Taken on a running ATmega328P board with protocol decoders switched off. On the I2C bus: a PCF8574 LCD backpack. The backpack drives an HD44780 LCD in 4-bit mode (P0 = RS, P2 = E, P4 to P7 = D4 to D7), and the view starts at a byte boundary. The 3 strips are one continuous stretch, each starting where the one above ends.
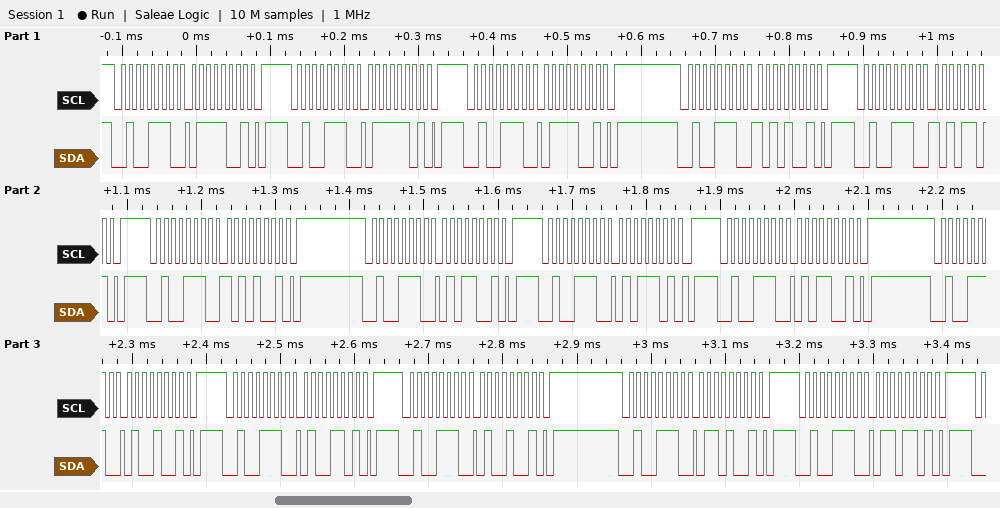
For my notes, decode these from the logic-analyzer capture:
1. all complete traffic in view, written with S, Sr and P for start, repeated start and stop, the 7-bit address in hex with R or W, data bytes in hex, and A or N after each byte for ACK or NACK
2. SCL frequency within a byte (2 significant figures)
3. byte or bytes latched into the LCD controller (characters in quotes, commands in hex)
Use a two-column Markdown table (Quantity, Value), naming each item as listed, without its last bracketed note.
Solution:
| Quantity | Value |
|---|---|
| all complete traffic in view, written with S, Sr and P for start, repeated start and stop, the 7-bit address in hex with R or W, data bytes in hex, and A or N after each byte for ACK or NACK | S 27W A 79 A P S 27W A 7D A P S 27W A 79 A P S 27W A A9 A P S 27W A AD A P S 27W A A9 A P S 27W A 59 A P S 27W A 5D A P S 27W A 59 A P S 27W A 49 A P S 27W A 4D A P S 27W A 49 A P S 27W A 69 A P S 27W A 6D A P |
| SCL frequency within a byte | 100 kHz |
| byte or bytes latched into the LCD controller | 'z' 'T' |
